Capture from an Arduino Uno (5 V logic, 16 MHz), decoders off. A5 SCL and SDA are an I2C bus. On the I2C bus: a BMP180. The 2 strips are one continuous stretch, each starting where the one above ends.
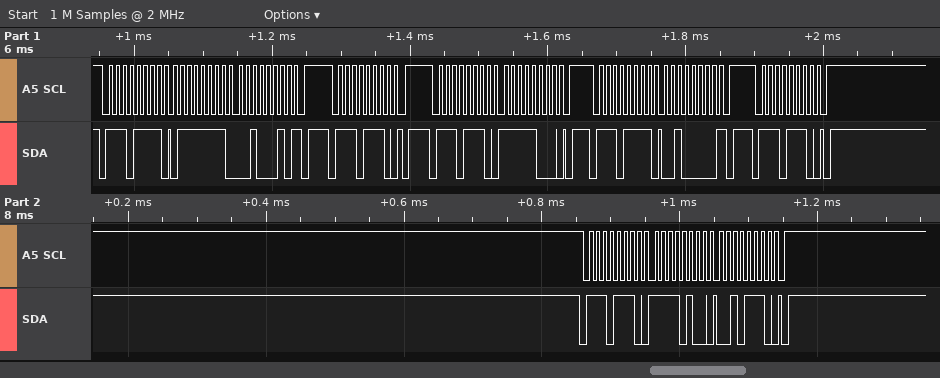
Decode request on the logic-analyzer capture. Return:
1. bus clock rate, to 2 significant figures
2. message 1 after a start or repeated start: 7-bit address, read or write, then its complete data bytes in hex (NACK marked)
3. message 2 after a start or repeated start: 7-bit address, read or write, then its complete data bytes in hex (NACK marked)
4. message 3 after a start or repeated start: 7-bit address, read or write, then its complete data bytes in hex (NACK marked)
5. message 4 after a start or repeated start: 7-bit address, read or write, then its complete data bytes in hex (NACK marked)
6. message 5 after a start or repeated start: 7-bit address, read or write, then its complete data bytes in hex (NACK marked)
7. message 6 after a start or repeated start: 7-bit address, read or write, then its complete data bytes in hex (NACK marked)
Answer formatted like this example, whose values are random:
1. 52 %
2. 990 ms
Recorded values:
1. 100 kHz
2. 0x77 read: 7F 22 NACK
3. 0x77 write
4. 0x77 write: F8
5. 0x77 read: 20 NACK
6. 0x77 write
7. 0x77 write: F4 2E
